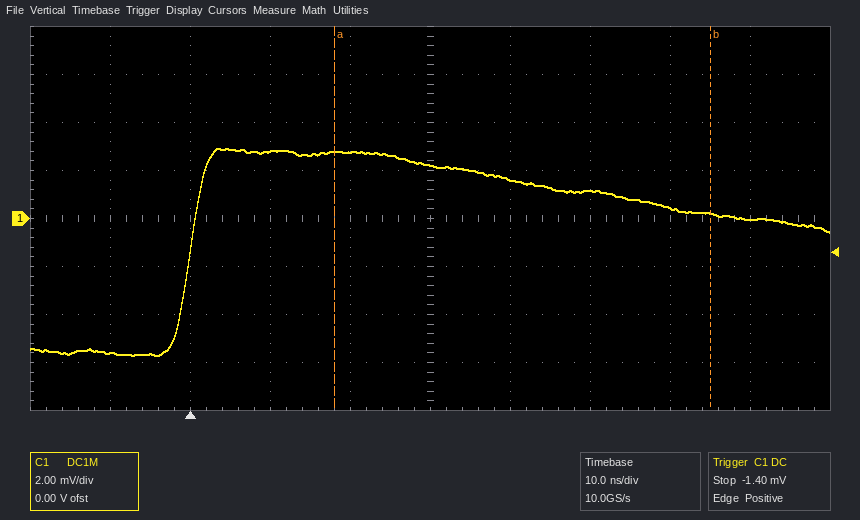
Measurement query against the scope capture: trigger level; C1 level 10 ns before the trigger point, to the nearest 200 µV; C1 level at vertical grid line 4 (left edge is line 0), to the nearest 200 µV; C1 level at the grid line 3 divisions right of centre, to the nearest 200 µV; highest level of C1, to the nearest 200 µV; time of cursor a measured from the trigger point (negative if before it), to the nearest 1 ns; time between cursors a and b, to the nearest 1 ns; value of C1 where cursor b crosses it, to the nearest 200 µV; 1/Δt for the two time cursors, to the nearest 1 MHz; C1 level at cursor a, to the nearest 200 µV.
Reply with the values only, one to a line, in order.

-1.40 mV
-5.6 mV
2.8 mV
400 µV
3.0 mV
+18 ns
47 ns
200 µV
21 MHz
2.8 mV
